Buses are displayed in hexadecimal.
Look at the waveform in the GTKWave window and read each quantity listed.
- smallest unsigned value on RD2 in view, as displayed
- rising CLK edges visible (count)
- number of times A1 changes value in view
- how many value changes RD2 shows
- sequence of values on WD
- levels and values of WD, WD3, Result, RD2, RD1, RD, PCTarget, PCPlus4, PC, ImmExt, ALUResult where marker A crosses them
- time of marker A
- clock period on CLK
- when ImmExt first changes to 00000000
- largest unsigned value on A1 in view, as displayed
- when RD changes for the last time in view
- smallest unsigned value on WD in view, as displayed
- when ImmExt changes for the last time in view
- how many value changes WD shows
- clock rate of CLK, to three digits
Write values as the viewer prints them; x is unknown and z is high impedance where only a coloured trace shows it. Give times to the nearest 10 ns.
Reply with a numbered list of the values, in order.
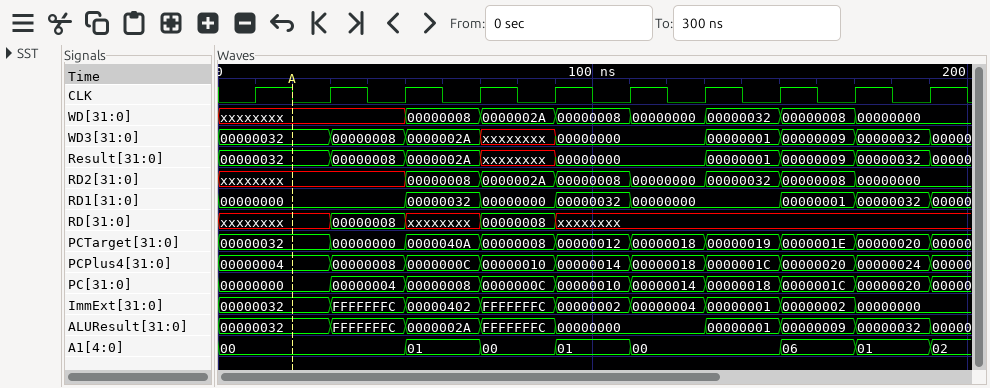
1. 00000000
2. 10
3. 7
4. 7
5. xxxxxxxx, 00000008, 0000002A, 00000008, 00000000, 00000032, 00000008, 00000000
6. WD=xxxxxxxx, WD3=00000032, Result=00000032, RD2=xxxxxxxx, RD1=00000000, RD=xxxxxxxx, PCTarget=00000032, PCPlus4=00000004, PC=00000000, ImmExt=00000032, ALUResult=00000032
7. 20 ns
8. 20 ns
9. 170 ns
10. 06
11. 90 ns
12. 00000000
13. 170 ns
14. 7
15. 50.0 MHz
